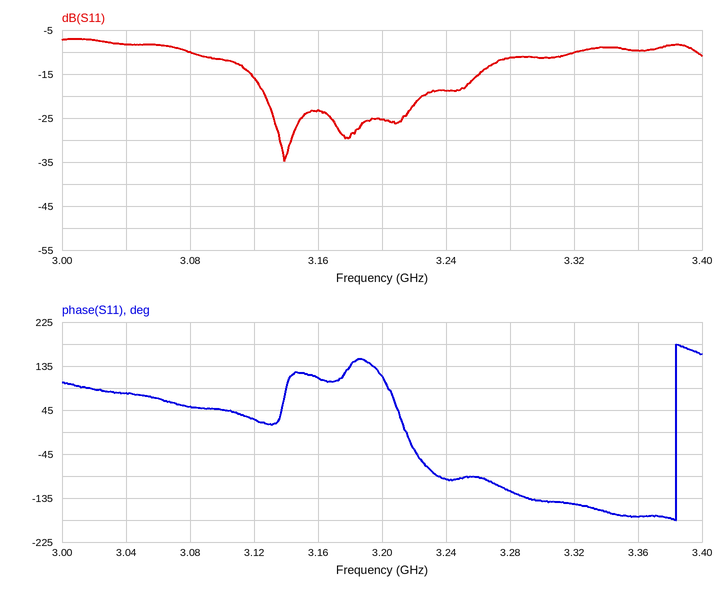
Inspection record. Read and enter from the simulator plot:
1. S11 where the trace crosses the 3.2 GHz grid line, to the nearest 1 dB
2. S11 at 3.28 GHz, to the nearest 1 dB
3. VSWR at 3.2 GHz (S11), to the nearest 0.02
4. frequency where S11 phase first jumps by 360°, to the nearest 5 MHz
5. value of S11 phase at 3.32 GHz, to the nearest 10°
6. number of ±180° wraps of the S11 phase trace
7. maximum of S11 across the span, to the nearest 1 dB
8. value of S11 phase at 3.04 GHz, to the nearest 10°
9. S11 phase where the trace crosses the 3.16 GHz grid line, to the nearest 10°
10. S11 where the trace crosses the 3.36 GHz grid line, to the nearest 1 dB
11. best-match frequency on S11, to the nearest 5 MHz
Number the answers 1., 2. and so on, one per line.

1. -25 dB
2. -11 dB
3. 1.12
4. 3.385 GHz
5. -150°
6. 1
7. -7 dB
8. 80°
9. 110°
10. -10 dB
11. 3.140 GHz
